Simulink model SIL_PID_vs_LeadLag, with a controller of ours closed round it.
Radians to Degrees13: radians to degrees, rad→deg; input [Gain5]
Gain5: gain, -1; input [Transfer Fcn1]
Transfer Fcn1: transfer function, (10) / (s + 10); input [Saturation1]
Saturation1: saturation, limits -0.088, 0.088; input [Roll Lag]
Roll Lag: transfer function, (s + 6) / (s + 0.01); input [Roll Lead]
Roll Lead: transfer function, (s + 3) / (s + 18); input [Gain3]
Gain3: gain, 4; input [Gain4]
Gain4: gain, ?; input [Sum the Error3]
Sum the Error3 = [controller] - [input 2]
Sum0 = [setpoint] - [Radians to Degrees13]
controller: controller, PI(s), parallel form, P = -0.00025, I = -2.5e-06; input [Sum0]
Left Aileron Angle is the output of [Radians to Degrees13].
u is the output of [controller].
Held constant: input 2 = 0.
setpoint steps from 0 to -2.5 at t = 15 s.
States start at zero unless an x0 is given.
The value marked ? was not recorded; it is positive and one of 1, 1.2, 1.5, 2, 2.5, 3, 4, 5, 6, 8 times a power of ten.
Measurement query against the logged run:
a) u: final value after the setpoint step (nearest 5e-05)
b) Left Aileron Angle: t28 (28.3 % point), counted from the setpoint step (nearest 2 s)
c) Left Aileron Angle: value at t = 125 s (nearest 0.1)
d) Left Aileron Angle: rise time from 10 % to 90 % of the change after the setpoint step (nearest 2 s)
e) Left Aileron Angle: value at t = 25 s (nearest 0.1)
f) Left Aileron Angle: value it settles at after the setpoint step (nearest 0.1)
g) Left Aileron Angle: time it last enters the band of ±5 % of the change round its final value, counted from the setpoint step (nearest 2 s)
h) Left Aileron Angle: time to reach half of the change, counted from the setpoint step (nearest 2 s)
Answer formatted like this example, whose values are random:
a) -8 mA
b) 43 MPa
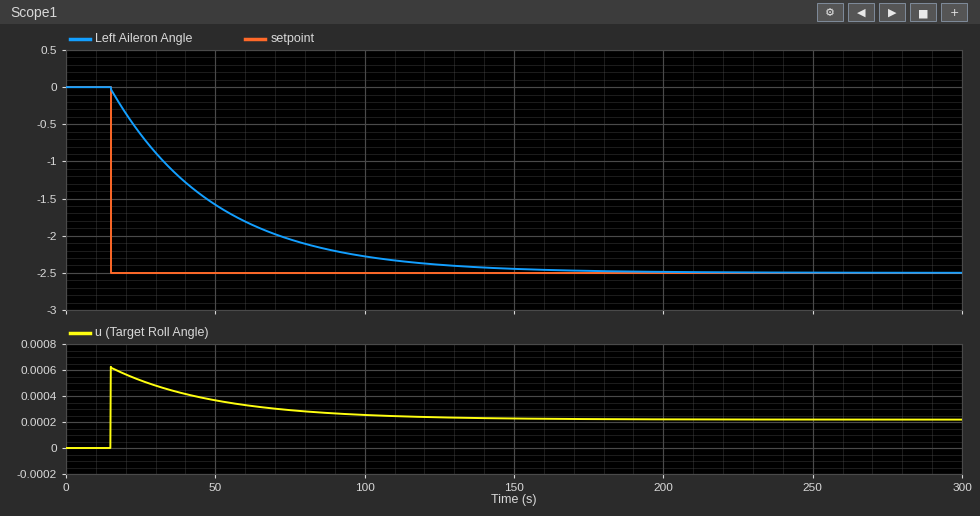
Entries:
a) 0.00020
b) 12 s
c) -2.4
d) 78 s
e) -0.6
f) -2.5
g) 106 s
h) 24 s
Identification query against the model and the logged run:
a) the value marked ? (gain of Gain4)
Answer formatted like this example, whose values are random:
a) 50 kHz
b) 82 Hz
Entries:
a) 0.5
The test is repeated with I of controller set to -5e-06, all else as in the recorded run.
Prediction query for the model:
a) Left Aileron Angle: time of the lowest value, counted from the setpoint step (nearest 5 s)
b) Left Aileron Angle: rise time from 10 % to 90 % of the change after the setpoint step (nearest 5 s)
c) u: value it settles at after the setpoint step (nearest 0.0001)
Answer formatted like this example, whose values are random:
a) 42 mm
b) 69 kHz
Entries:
a) 115 s
b) 50 s
c) 0.0002
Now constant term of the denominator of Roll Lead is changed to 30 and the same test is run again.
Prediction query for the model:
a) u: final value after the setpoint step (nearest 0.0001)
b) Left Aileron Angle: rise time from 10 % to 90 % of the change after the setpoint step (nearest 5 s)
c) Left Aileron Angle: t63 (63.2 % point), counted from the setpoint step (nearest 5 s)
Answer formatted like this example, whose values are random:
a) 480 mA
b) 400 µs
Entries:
a) 0.0004
b) 130 s
c) 60 s
